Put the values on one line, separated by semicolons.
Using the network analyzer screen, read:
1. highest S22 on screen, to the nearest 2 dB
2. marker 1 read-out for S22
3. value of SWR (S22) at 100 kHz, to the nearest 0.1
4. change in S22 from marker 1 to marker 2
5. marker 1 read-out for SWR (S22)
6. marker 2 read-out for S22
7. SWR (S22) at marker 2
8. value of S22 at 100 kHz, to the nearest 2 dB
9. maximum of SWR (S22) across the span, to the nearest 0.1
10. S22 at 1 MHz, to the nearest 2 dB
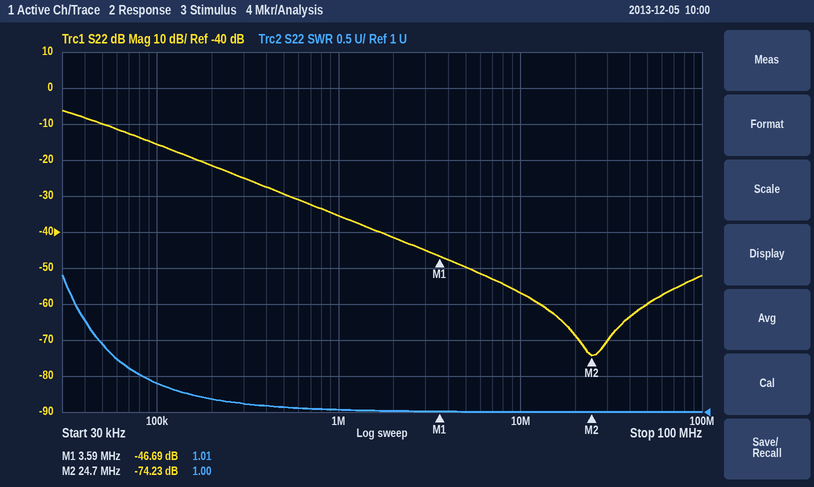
-6 dB; -46.69 dB; 1.4; -27.54 dB; 1.01; -74.23 dB; 1.00; -16 dB; 2.9; -36 dB
